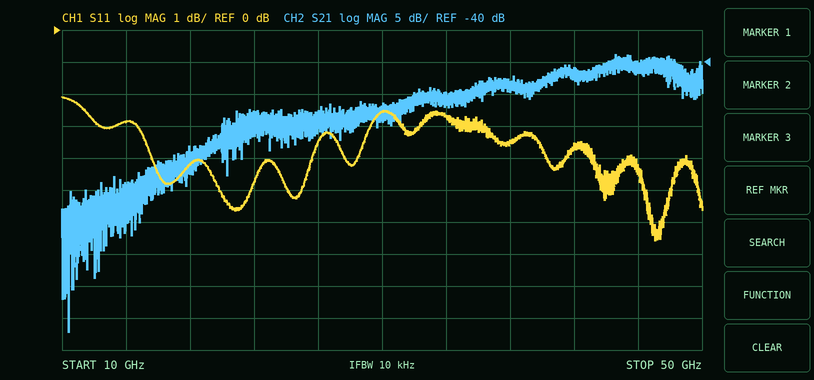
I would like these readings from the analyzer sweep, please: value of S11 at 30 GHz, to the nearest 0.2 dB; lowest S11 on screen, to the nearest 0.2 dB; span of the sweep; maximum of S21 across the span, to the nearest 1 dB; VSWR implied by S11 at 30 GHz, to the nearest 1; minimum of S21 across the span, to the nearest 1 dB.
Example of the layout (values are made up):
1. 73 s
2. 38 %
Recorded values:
1. -2.6 dB
2. -6.6 dB
3. 40 GHz
4. -39 dB
5. 7
6. -82 dB
